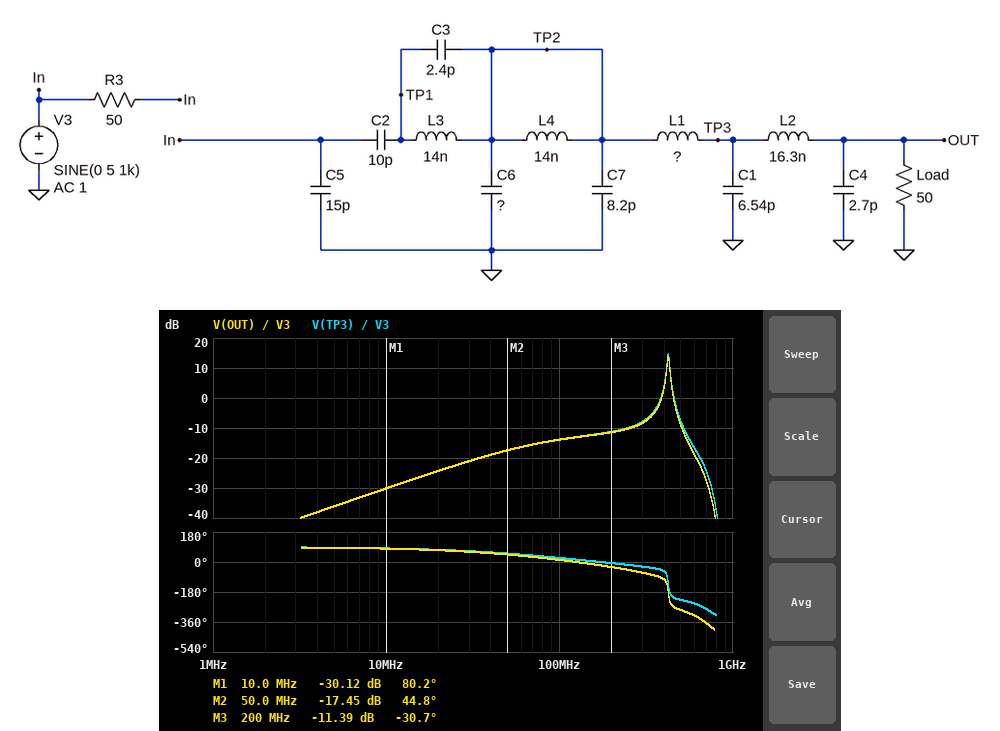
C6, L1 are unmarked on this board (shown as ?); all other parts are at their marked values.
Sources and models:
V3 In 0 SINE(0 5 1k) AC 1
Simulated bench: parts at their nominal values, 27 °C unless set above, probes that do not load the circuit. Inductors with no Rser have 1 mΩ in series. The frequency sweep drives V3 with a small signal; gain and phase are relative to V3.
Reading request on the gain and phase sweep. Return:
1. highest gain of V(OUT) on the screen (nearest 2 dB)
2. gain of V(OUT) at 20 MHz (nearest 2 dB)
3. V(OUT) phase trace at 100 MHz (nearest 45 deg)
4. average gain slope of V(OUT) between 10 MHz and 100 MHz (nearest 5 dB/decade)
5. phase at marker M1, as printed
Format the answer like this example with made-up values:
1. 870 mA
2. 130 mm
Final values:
1. 14 dB
2. -24 dB
3. 0 deg
4. 15 dB/decade
5. 80.2 deg
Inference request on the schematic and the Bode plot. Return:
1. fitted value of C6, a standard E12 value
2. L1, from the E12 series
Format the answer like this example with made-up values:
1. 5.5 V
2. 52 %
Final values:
1. 27 pF
2. 18 nH
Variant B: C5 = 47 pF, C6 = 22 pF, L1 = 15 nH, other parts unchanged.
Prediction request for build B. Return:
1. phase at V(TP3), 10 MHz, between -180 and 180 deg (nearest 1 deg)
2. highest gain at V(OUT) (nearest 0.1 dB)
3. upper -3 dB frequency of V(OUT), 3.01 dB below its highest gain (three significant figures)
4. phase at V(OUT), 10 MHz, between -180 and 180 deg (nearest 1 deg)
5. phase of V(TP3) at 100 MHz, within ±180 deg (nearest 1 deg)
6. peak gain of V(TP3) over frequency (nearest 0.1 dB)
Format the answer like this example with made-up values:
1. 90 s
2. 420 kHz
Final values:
1. 82 deg
2. 12.3 dB
3. 438 MHz
4. 81 deg
5. 29 deg
6. 13.2 dB
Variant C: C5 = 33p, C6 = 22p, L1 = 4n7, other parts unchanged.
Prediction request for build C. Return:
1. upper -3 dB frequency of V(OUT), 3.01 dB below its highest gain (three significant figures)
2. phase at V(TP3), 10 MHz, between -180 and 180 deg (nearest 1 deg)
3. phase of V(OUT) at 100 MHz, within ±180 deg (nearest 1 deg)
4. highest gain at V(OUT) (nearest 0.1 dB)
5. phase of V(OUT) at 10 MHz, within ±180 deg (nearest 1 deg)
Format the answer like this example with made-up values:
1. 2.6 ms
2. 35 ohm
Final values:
1. 432 MHz
2. 82 deg
3. 22 deg
4. 13.0 dB
5. 81 deg
